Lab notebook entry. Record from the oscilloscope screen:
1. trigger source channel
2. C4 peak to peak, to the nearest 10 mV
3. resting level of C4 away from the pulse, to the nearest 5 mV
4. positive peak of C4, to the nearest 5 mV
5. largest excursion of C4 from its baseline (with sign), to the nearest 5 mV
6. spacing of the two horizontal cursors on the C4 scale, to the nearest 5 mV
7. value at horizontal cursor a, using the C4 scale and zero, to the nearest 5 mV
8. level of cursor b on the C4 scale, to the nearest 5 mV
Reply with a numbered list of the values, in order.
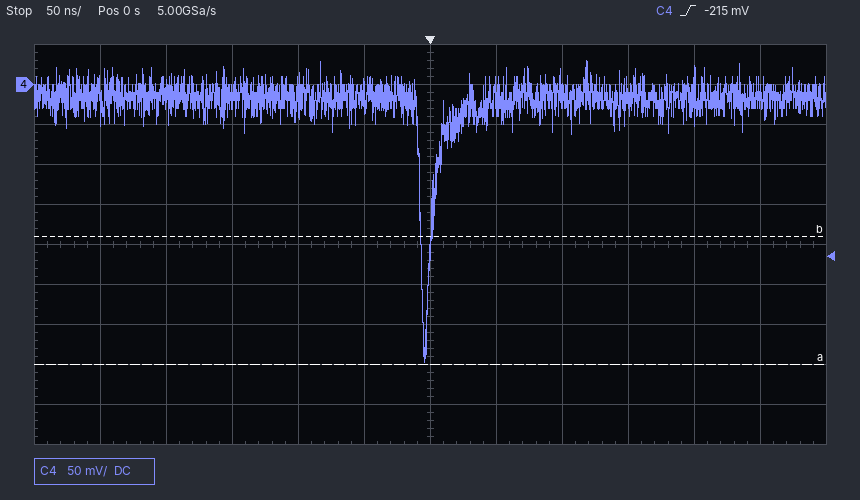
1. C4
2. 380 mV
3. -15 mV
4. 30 mV
5. -330 mV
6. 160 mV
7. -350 mV
8. -190 mV
